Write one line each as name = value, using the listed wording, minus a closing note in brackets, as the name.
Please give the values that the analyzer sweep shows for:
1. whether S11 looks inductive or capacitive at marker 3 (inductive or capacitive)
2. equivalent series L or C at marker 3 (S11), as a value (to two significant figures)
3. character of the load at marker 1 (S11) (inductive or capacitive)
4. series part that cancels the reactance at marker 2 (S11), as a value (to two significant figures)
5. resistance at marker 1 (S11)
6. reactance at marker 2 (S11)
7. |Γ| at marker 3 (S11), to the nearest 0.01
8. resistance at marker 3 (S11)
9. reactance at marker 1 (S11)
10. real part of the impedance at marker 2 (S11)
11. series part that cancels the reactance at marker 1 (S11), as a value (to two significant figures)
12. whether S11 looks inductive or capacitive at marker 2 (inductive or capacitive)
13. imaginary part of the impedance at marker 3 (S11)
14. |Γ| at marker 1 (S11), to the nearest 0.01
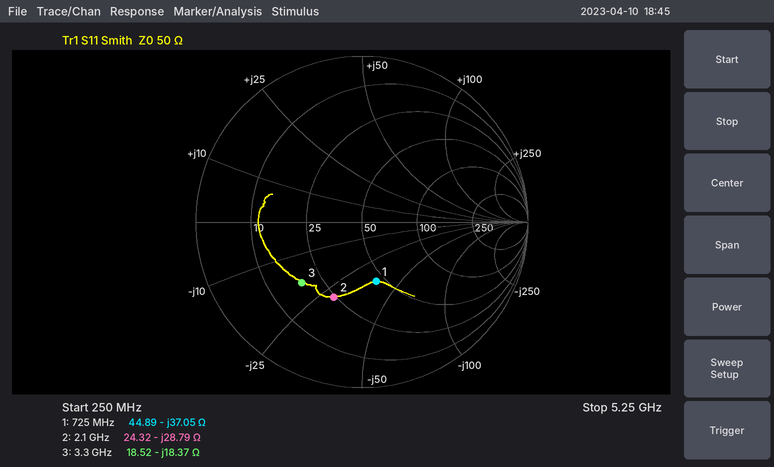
whether S11 looks inductive or capacitive at marker 3 = capacitive
equivalent series L or C at marker 3 (S11), as a value = 2.6 pF
character of the load at marker 1 (S11) = capacitive
series part that cancels the reactance at marker 2 (S11), as a value = 2.2 nH
resistance at marker 1 = 44.89 Ω
reactance at marker 2 = -28.79 Ω
|Γ| at marker 3 (S11), to the nearest 0.01 = 0.51
resistance at marker 3 = 18.52 Ω
reactance at marker 1 = -37.05 Ω
real part of the impedance at marker 2 = 24.32 Ω
series part that cancels the reactance at marker 1 (S11), as a value = 8.1 nH
whether S11 looks inductive or capacitive at marker 2 = capacitive
imaginary part of the impedance at marker 3 = -18.37 Ω
|Γ| at marker 1 (S11), to the nearest 0.01 = 0.37
